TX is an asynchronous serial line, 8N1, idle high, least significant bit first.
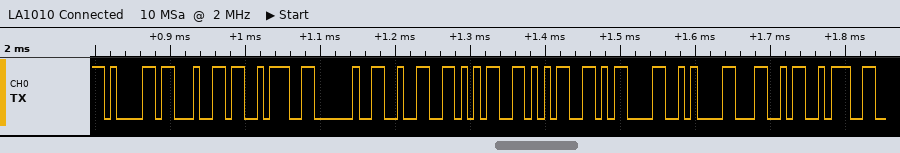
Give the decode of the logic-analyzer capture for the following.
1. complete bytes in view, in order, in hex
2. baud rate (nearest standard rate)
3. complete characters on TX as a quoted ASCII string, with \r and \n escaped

61 64 3A 20 32 35 35 0D 0A 4C 3A
115200 baud
"ad: 255\r\nL:"
